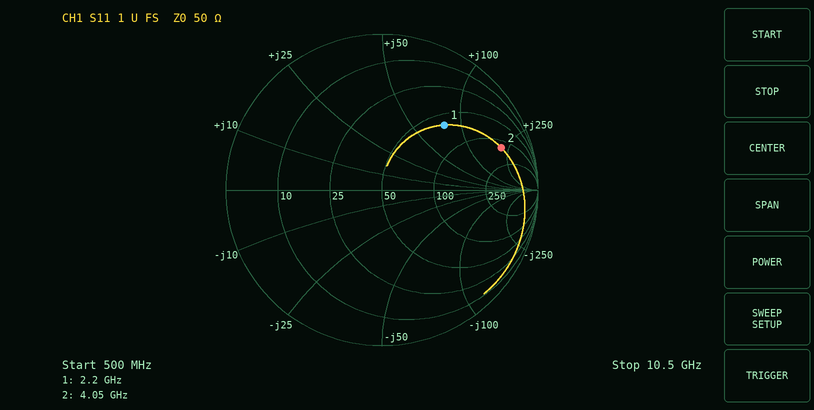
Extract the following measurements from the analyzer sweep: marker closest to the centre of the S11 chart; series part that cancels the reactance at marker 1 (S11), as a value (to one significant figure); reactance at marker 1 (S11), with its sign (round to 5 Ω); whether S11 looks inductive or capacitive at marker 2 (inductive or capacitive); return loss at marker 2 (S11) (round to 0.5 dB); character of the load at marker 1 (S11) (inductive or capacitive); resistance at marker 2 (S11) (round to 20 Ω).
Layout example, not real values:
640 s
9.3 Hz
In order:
marker 1
900 fF
+80 Ω
inductive
2.0 dB
inductive
140 Ω
